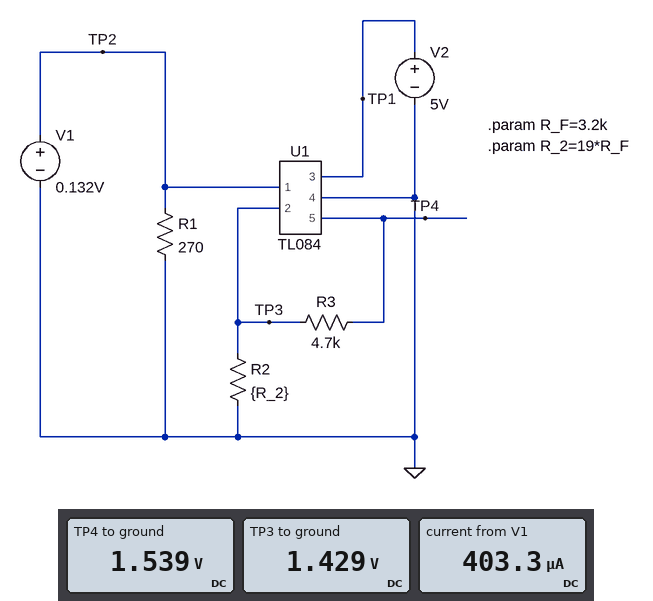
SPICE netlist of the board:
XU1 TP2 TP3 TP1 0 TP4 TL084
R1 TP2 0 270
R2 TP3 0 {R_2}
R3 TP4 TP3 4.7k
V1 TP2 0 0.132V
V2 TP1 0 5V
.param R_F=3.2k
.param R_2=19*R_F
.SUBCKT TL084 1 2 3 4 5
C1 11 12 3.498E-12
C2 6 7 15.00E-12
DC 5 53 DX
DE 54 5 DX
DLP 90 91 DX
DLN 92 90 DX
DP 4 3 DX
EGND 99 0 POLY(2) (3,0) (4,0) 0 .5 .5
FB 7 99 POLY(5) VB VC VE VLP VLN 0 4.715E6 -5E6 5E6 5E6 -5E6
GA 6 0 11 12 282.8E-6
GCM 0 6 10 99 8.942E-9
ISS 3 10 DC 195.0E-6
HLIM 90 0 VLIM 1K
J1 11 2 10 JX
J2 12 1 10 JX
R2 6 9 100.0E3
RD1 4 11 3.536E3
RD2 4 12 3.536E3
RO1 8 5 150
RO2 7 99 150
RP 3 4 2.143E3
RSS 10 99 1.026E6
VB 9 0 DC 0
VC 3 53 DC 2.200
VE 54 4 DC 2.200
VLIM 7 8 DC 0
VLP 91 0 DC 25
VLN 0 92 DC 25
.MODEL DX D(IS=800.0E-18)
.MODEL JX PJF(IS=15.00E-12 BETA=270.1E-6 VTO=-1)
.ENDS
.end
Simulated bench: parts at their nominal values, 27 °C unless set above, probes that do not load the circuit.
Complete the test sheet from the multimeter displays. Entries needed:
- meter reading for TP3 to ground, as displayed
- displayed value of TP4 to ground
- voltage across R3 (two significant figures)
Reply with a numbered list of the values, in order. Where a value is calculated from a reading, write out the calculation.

1. 1.429 V
2. 1.539 V
3. 1.539 V - 1.429 V = 110 mV
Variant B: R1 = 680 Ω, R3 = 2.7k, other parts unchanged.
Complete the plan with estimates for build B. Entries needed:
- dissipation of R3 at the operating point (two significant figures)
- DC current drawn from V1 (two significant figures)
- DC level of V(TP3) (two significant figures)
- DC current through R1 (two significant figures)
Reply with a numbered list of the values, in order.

1. 1.6 µW
2. 110 µA
3. 1.5 V
4. 190 µA
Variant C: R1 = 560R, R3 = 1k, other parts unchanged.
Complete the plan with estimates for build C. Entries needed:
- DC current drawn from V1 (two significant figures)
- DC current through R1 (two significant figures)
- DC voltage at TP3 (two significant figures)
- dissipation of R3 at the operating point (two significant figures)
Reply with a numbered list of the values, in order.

1. 150 µA
2. 240 µA
3. 1.5 V
4. 620 nW
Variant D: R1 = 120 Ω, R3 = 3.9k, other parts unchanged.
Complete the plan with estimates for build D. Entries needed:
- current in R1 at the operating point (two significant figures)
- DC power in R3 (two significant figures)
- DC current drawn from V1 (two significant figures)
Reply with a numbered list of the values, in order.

1. 1.1 mA
2. 2.2 µW
3. 1.0 mA
